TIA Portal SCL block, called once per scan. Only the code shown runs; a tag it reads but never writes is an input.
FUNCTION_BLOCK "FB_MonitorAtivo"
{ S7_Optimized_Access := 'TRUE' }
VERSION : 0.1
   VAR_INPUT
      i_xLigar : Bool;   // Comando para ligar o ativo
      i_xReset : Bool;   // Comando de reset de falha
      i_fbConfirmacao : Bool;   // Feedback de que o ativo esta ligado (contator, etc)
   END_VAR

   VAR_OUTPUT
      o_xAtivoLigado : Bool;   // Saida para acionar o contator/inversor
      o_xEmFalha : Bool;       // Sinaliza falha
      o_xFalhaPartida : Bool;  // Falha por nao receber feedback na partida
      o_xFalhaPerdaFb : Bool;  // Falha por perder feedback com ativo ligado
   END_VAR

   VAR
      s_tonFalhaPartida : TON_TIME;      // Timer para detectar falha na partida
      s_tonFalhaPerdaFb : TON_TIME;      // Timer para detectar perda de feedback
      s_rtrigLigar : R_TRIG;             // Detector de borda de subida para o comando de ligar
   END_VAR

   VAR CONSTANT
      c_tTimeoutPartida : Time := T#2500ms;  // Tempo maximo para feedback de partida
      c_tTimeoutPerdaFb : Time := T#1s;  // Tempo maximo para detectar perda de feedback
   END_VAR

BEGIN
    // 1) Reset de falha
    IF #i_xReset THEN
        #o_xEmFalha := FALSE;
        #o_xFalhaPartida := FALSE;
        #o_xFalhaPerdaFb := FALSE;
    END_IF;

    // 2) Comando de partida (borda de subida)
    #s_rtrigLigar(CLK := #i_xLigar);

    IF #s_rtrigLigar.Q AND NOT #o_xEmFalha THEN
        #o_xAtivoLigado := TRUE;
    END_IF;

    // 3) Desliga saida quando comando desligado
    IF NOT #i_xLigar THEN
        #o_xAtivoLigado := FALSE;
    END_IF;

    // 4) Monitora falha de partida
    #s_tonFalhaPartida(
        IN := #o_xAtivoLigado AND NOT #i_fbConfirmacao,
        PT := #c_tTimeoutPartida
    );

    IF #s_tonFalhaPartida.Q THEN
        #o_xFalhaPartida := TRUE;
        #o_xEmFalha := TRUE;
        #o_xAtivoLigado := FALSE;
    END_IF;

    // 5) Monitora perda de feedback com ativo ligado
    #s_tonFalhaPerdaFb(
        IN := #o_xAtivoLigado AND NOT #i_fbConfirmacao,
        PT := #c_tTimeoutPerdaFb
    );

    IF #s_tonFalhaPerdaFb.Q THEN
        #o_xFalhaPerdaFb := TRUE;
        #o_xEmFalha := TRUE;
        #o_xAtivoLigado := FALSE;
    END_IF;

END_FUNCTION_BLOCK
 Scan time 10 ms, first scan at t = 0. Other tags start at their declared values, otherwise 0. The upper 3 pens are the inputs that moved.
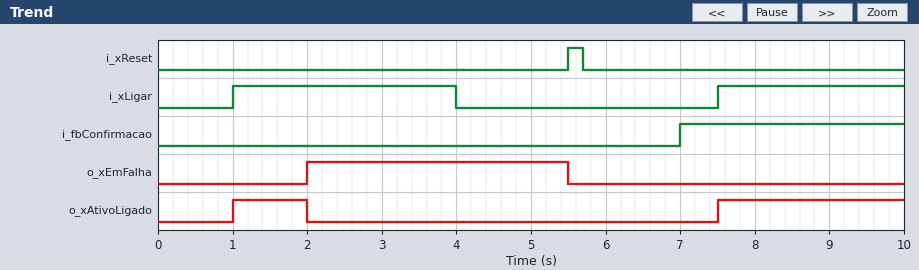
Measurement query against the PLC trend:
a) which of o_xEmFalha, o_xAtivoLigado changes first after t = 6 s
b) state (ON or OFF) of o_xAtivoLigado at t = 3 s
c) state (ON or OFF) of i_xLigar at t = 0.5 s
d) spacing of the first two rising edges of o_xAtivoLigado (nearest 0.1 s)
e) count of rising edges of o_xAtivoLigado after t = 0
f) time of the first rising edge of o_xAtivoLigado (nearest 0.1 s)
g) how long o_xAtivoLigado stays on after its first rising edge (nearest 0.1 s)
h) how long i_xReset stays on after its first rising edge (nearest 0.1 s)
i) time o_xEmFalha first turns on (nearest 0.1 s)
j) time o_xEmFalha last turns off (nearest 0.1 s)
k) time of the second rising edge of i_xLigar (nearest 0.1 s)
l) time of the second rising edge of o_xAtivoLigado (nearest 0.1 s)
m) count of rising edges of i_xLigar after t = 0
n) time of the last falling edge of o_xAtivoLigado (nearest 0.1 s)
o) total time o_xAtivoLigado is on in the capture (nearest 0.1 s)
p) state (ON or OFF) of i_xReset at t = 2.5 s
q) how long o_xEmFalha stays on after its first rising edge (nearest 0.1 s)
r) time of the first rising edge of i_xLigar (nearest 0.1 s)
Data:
o_xAtivoLigado
OFF
OFF
6.5 s
2
1.0 s
1.0 s
0.2 s
2.0 s
5.5 s
7.5 s
7.5 s
2
2.0 s
3.5 s
OFF
3.5 s
1.0 s
